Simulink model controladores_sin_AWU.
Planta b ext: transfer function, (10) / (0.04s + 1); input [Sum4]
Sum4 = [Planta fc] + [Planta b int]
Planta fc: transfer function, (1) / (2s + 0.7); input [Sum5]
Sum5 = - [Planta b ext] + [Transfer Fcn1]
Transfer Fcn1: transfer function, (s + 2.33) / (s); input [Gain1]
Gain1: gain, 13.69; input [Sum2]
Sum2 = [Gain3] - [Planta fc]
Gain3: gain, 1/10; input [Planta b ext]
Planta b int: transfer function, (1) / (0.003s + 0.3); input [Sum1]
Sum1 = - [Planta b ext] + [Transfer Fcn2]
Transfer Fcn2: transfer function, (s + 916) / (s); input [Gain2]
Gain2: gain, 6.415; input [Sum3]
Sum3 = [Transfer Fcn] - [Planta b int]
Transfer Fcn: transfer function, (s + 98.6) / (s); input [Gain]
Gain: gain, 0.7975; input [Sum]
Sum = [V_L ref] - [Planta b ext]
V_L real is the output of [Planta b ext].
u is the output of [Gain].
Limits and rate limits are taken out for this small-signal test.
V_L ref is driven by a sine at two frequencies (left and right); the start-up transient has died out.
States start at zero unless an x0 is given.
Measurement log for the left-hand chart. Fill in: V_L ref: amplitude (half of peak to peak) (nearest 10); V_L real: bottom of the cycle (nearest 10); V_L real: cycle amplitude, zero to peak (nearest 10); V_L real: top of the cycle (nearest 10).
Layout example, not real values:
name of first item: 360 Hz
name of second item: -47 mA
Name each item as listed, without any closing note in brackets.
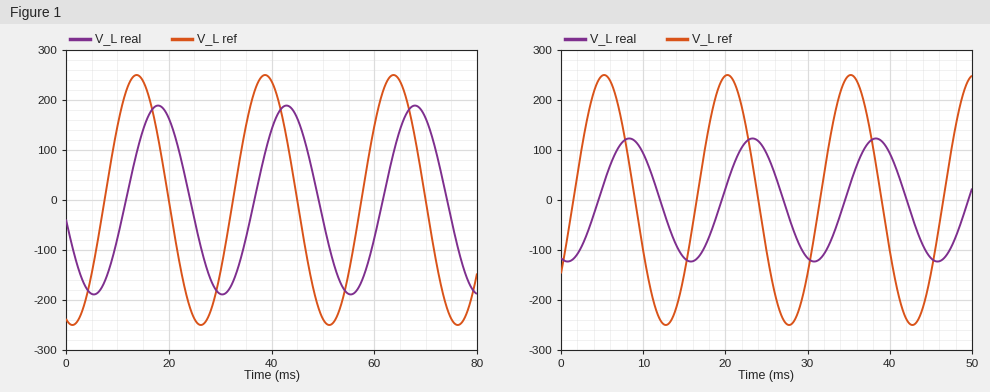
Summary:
V_L ref: amplitude (half of peak to peak): 250
V_L real: bottom of the cycle: -190
V_L real: cycle amplitude, zero to peak: 190
V_L real: top of the cycle: 190
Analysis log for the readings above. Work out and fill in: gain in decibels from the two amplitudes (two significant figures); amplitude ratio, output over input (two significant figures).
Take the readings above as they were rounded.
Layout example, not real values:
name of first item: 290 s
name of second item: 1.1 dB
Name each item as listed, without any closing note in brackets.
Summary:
gain in decibels from the two amplitudes: -2.4 dB
amplitude ratio, output over input: 0.76
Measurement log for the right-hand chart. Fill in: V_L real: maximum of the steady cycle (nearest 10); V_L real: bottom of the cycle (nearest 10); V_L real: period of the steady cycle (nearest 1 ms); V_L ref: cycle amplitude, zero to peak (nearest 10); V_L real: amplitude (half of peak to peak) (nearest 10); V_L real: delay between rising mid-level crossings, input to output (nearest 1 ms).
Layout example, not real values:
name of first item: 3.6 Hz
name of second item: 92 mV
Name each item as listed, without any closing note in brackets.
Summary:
V_L real: maximum of the steady cycle: 120
V_L real: bottom of the cycle: -120
V_L real: period of the steady cycle: 15 ms
V_L ref: cycle amplitude, zero to peak: 250
V_L real: amplitude (half of peak to peak): 120
V_L real: delay between rising mid-level crossings, input to output: 3 ms
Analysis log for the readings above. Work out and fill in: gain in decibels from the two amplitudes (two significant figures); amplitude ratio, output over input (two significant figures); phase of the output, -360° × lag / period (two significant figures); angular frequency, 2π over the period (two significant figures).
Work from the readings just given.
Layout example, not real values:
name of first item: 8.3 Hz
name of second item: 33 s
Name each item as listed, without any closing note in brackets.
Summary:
gain in decibels from the two amplitudes: -6.4 dB
amplitude ratio, output over input: 0.48
phase of the output, -360° × lag / period: -72°
angular frequency, 2π over the period: 0.42 rad/ms
